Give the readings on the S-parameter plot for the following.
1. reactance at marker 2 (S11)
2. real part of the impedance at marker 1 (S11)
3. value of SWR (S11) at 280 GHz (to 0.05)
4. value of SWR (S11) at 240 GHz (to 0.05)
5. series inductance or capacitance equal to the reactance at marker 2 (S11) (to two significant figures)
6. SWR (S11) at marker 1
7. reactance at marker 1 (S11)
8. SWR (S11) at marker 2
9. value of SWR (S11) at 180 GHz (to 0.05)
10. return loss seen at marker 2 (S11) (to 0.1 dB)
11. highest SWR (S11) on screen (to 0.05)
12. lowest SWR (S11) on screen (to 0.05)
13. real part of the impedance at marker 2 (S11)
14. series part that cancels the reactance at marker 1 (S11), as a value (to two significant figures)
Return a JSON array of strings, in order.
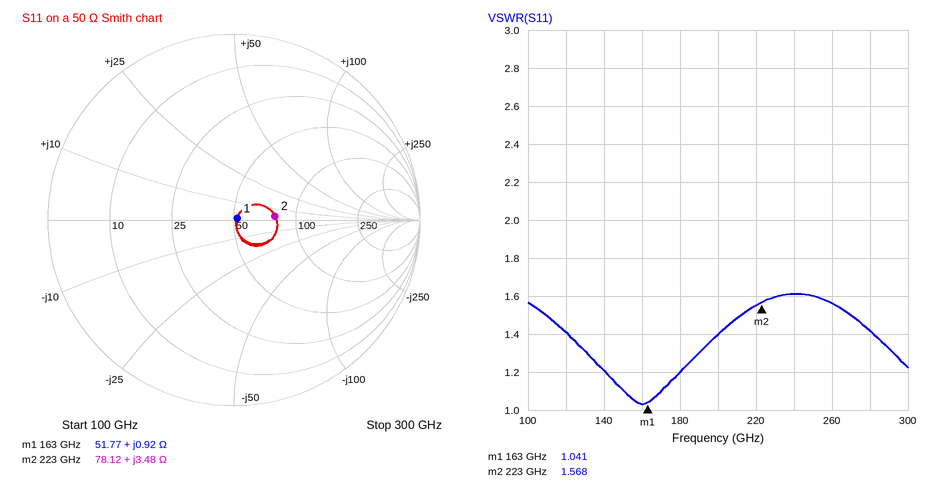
["+3.48 Ω", "51.77 Ω", "1.40", "1.60", "2.5 pH", "1.041", "+0.92 Ω", "1.568", "1.20", "13.1 dB", "1.60", "1.05", "78.12 Ω", "1.1 pF"]
